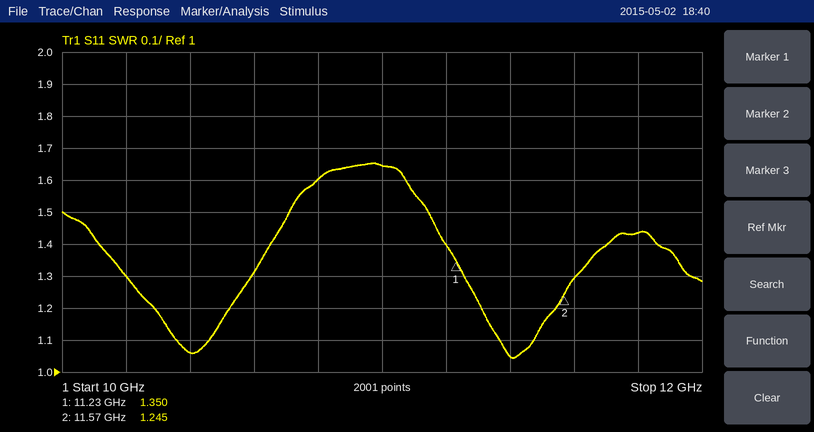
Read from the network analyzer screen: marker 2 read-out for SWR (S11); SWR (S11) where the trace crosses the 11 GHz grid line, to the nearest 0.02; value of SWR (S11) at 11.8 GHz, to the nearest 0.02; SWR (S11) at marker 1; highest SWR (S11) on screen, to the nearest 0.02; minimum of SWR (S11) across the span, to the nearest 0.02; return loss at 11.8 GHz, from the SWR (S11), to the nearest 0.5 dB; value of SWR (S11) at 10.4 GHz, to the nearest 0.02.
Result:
1.245
1.64
1.44
1.350
1.66
1.04
15.0 dB
1.06
